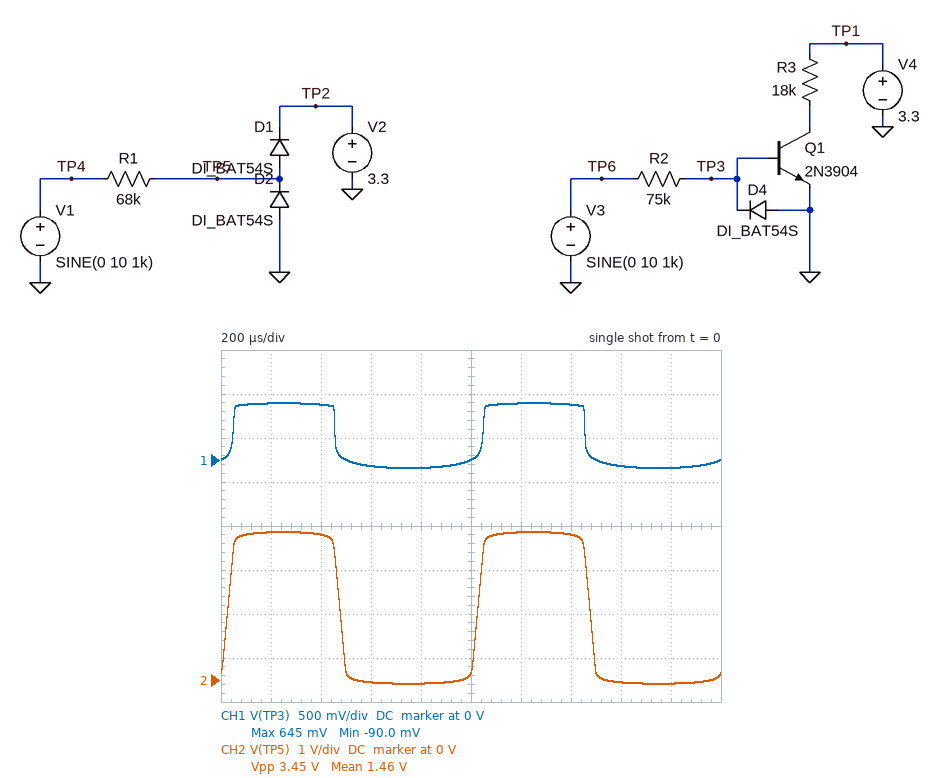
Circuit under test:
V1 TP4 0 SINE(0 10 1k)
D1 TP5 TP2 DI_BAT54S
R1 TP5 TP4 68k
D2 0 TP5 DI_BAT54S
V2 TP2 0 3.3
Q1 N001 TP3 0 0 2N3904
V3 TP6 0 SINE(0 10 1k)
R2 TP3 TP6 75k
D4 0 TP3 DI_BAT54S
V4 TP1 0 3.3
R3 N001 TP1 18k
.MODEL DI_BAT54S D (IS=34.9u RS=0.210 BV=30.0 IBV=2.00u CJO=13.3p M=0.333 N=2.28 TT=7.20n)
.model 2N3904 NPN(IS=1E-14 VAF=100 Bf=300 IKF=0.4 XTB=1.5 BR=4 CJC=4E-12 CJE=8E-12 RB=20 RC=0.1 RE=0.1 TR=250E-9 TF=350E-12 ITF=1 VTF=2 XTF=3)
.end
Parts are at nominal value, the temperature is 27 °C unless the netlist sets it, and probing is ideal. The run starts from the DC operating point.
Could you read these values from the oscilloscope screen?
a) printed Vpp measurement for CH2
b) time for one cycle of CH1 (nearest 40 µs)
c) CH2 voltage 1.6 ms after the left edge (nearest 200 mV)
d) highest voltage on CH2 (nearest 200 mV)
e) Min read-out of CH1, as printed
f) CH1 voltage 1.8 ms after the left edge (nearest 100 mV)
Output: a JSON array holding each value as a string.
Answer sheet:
["3.45 V", "1.00 ms", "0 V", "3.4 V", "-90.0 mV", "-100 mV"]
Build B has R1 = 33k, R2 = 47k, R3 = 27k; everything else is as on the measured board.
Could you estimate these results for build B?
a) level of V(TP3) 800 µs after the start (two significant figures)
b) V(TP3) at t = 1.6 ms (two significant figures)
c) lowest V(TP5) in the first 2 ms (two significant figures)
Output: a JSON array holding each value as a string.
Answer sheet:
["-110 mV", "-89 mV", "-130 mV"]
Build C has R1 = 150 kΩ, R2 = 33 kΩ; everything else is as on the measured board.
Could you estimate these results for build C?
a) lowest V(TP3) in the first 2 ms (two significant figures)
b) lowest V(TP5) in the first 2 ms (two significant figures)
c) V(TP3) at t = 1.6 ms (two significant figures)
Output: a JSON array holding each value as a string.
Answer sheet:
["-130 mV", "-38 mV", "-110 mV"]
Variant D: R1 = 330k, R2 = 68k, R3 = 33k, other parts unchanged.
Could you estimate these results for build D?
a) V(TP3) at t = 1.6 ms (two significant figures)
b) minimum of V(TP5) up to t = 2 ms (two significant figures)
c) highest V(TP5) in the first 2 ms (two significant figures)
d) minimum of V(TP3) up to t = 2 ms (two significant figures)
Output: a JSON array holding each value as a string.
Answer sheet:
["-73 mV", "8.3 mV", "3.3 V", "-97 mV"]
